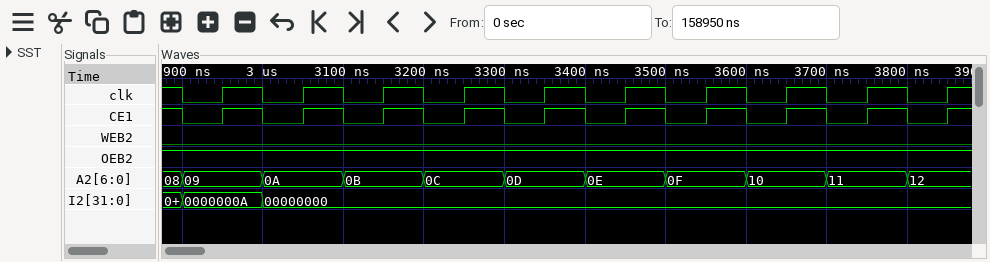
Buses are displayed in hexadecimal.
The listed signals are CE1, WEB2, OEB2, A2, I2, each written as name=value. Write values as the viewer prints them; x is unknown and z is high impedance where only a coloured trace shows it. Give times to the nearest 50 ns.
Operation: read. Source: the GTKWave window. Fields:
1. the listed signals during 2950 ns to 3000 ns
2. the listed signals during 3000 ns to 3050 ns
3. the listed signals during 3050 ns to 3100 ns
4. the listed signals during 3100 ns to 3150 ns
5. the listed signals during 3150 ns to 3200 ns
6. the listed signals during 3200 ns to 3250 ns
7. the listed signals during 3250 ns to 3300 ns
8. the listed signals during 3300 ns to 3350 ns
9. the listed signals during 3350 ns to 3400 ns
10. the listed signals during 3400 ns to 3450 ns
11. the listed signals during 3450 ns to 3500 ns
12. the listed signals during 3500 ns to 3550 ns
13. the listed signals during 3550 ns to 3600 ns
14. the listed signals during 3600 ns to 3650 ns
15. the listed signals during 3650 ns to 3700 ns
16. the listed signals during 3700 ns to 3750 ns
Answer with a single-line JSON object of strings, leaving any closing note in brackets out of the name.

{"the listed signals during 2950 ns to 3000 ns": "CE1=1, WEB2=0, OEB2=1, A2=09, I2=0000000A", "the listed signals during 3000 ns to 3050 ns": "CE1=0, WEB2=0, OEB2=1, A2=0A, I2=00000000", "the listed signals during 3050 ns to 3100 ns": "CE1=1, WEB2=0, OEB2=1, A2=0A, I2=00000000", "the listed signals during 3100 ns to 3150 ns": "CE1=0, WEB2=0, OEB2=1, A2=0B, I2=00000000", "the listed signals during 3150 ns to 3200 ns": "CE1=1, WEB2=0, OEB2=1, A2=0B, I2=00000000", "the listed signals during 3200 ns to 3250 ns": "CE1=0, WEB2=0, OEB2=1, A2=0C, I2=00000000", "the listed signals during 3250 ns to 3300 ns": "CE1=1, WEB2=0, OEB2=1, A2=0C, I2=00000000", "the listed signals during 3300 ns to 3350 ns": "CE1=0, WEB2=0, OEB2=1, A2=0D, I2=00000000", "the listed signals during 3350 ns to 3400 ns": "CE1=1, WEB2=0, OEB2=1, A2=0D, I2=00000000", "the listed signals during 3400 ns to 3450 ns": "CE1=0, WEB2=0, OEB2=1, A2=0E, I2=00000000", "the listed signals during 3450 ns to 3500 ns": "CE1=1, WEB2=0, OEB2=1, A2=0E, I2=00000000", "the listed signals during 3500 ns to 3550 ns": "CE1=0, WEB2=0, OEB2=1, A2=0F, I2=00000000", "the listed signals during 3550 ns to 3600 ns": "CE1=1, WEB2=0, OEB2=1, A2=0F, I2=00000000", "the listed signals during 3600 ns to 3650 ns": "CE1=0, WEB2=0, OEB2=1, A2=10, I2=00000000", "the listed signals during 3650 ns to 3700 ns": "CE1=1, WEB2=0, OEB2=1, A2=10, I2=00000000", "the listed signals during 3700 ns to 3750 ns": "CE1=0, WEB2=0, OEB2=1, A2=11, I2=00000000"}
